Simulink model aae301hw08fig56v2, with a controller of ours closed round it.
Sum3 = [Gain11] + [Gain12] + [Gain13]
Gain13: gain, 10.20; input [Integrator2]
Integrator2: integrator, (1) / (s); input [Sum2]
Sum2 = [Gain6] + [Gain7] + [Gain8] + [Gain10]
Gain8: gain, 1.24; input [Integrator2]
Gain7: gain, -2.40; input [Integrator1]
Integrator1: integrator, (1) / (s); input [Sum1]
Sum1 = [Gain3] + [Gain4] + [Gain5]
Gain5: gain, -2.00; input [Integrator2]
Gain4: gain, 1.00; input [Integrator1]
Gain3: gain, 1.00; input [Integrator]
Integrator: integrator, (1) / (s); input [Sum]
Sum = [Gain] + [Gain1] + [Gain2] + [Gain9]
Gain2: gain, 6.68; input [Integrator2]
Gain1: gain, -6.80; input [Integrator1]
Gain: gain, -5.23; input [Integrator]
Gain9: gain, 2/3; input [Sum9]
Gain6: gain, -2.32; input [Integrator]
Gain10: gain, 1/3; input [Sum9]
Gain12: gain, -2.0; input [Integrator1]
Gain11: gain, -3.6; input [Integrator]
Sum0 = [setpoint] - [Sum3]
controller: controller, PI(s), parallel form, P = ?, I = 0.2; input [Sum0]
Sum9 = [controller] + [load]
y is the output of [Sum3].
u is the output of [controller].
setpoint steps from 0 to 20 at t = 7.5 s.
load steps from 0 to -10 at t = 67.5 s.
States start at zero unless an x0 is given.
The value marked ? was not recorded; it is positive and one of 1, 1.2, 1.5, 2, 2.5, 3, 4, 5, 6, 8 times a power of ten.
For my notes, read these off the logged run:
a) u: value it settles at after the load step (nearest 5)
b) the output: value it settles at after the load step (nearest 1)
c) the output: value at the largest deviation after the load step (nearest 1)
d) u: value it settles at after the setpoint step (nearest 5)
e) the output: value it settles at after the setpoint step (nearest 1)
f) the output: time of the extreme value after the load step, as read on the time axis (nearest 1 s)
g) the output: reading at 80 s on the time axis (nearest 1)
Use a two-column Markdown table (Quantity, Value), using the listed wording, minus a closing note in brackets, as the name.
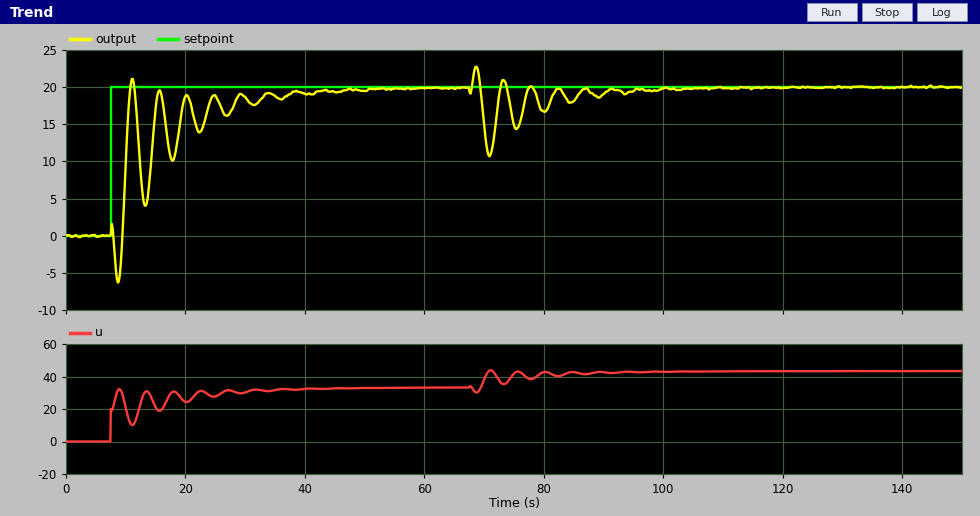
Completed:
| Quantity | Value |
|---|---|
| u: value it settles at after the load step | 45 |
| the output: value it settles at after the load step | 20 |
| the output: value at the largest deviation after the load step | 11 |
| u: value it settles at after the setpoint step | 35 |
| the output: value it settles at after the setpoint step | 20 |
| the output: time of the extreme value after the load step, as read on the time axis | 71 s |
| the output: reading at 80 s on the time axis | 17 |
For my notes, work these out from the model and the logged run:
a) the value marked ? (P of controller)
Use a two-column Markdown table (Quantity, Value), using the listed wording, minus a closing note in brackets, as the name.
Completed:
| Quantity | Value |
|---|---|
| the value marked ? | 1 |
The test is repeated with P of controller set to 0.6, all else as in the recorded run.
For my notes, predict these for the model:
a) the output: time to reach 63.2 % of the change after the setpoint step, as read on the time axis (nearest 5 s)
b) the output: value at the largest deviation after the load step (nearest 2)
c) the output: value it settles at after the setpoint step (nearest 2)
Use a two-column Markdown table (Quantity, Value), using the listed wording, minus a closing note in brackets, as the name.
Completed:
| Quantity | Value |
|---|---|
| the output: time to reach 63.2 % of the change after the setpoint step, as read on the time axis | 15 s |
| the output: value at the largest deviation after the load step | 12 |
| the output: value it settles at after the setpoint step | 20 |
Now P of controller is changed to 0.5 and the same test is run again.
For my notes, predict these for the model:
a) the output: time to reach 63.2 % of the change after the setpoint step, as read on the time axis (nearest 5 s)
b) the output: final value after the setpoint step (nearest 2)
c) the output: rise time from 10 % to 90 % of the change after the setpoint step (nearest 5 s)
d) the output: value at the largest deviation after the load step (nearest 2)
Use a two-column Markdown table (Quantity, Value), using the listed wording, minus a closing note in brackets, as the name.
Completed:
| Quantity | Value |
|---|---|
| the output: time to reach 63.2 % of the change after the setpoint step, as read on the time axis | 15 s |
| the output: final value after the setpoint step | 20 |
| the output: rise time from 10 % to 90 % of the change after the setpoint step | 15 s |
| the output: value at the largest deviation after the load step | 12 |
